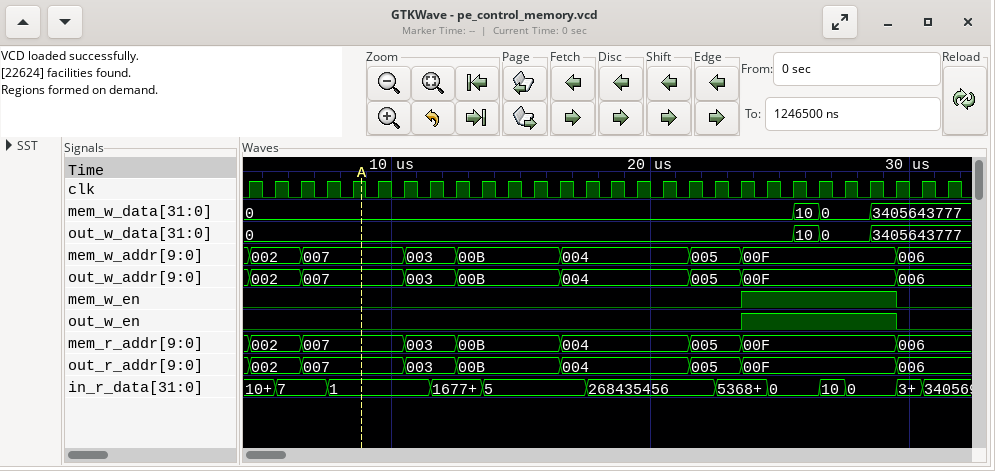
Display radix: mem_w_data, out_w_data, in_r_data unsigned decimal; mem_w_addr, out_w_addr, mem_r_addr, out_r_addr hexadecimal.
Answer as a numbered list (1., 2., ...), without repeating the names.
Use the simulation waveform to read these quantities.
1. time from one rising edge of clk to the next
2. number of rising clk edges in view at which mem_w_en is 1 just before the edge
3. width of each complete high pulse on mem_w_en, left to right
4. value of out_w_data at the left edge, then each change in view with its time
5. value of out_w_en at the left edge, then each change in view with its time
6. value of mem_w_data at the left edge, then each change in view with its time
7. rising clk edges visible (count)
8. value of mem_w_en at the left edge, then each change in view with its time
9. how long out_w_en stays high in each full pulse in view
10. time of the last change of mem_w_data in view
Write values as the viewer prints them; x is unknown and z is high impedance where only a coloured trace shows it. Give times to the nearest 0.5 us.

1. 1 us
2. 6
3. 6 us
4. 0, 10 at 25.5 us, 0 at 26.5 us, 3405643777 at 28.5 us
5. 0, 1 at 23.5 us, 0 at 29.5 us
6. 0, 10 at 25.5 us, 0 at 26.5 us, 3405643777 at 28.5 us
7. 28
8. 0, 1 at 23.5 us, 0 at 29.5 us
9. 6 us
10. 28.5 us
